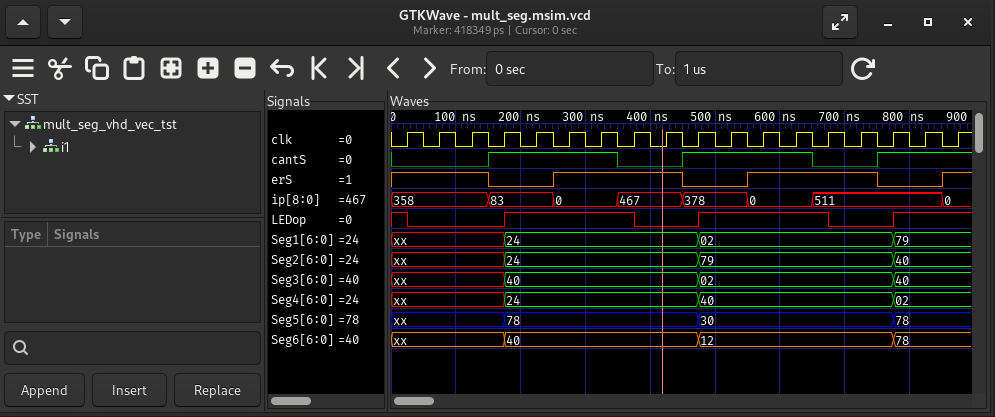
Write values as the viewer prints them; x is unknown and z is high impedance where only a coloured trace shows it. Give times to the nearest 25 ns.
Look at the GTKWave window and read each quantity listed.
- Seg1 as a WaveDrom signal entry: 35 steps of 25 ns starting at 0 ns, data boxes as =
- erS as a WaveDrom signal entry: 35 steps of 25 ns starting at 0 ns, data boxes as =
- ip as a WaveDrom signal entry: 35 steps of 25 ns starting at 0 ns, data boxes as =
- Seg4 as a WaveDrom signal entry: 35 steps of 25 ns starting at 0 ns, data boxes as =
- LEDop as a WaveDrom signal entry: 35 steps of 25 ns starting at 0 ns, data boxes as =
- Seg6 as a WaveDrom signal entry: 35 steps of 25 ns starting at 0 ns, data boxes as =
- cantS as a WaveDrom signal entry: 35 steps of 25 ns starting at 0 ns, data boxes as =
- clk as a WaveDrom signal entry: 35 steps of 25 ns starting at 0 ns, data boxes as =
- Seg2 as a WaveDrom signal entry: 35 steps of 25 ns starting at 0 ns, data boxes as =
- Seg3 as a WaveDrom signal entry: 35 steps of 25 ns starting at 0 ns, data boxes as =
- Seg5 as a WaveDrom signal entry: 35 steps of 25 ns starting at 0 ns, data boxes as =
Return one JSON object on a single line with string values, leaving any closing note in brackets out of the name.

{"Seg1 as a WaveDrom signal entry: 35 steps of 25 ns starting at 0 ns, data boxes as =": "{name: 'Seg1', wave: 'x......=...........=...........=...', data: '24 02 79'}", "erS as a WaveDrom signal entry: 35 steps of 25 ns starting at 0 ns, data boxes as =": "{name: 'erS', wave: '1.....0...1.......0...1.......0...1'}", "ip as a WaveDrom signal entry: 35 steps of 25 ns starting at 0 ns, data boxes as =": "{name: 'ip', wave: '=.....=...=...=...=...=...=.......=', data: '358 83 0 467 378 0 511 0'}", "Seg4 as a WaveDrom signal entry: 35 steps of 25 ns starting at 0 ns, data boxes as =": "{name: 'Seg4', wave: 'x......=...........=...........=...', data: '24 40 02'}", "LEDop as a WaveDrom signal entry: 35 steps of 25 ns starting at 0 ns, data boxes as =": "{name: 'LEDop', wave: '10.....1.......0...1.......0...1...'}", "Seg6 as a WaveDrom signal entry: 35 steps of 25 ns starting at 0 ns, data boxes as =": "{name: 'Seg6', wave: 'x......=...........=...........=...', data: '40 12 78'}", "cantS as a WaveDrom signal entry: 35 steps of 25 ns starting at 0 ns, data boxes as =": "{name: 'cantS', wave: '0.....1.......0...1.......0...1....'}", "clk as a WaveDrom signal entry: 35 steps of 25 ns starting at 0 ns, data boxes as =": "{name: 'clk', wave: '01010101010101010101010101010101010'}", "Seg2 as a WaveDrom signal entry: 35 steps of 25 ns starting at 0 ns, data boxes as =": "{name: 'Seg2', wave: 'x......=...........=...........=...', data: '24 79 40'}", "Seg3 as a WaveDrom signal entry: 35 steps of 25 ns starting at 0 ns, data boxes as =": "{name: 'Seg3', wave: 'x......=...........=...........=...', data: '40 02 40'}", "Seg5 as a WaveDrom signal entry: 35 steps of 25 ns starting at 0 ns, data boxes as =": "{name: 'Seg5', wave: 'x......=...........=...........=...', data: '78 30 78'}"}
